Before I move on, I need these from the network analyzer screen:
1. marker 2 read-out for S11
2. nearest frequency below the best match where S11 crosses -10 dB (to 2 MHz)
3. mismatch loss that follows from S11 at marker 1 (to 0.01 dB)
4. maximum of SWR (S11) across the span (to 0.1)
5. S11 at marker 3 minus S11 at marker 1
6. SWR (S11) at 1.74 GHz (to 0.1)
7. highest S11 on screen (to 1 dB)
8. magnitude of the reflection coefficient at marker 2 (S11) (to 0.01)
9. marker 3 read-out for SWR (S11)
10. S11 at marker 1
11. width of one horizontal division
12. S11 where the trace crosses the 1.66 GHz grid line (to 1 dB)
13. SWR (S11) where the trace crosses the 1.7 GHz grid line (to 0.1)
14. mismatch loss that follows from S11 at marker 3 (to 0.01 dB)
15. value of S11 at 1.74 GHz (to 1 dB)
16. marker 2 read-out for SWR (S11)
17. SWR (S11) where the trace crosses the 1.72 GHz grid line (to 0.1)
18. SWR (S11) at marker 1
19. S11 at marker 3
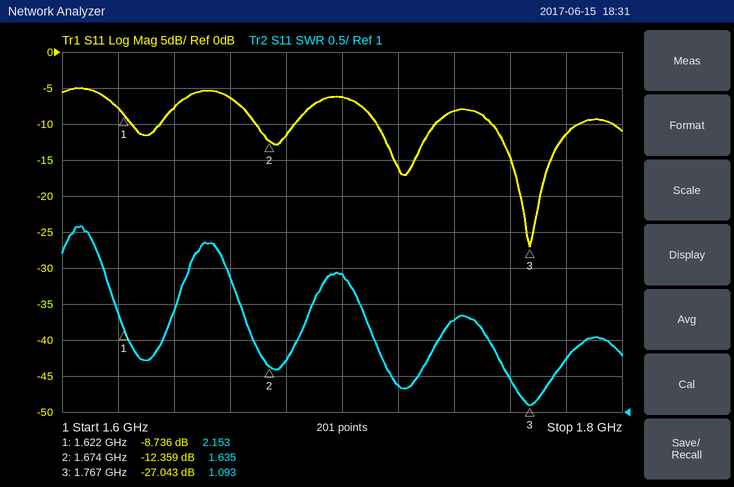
-12.359 dB
1.754 GHz
0.62 dB
3.6
-18.307 dB
2.3
-5 dB
0.24
1.093
-8.736 dB
20 MHz
-6 dB
2.9
0.01 dB
-8 dB
1.635
1.4
2.153
-27.043 dB
